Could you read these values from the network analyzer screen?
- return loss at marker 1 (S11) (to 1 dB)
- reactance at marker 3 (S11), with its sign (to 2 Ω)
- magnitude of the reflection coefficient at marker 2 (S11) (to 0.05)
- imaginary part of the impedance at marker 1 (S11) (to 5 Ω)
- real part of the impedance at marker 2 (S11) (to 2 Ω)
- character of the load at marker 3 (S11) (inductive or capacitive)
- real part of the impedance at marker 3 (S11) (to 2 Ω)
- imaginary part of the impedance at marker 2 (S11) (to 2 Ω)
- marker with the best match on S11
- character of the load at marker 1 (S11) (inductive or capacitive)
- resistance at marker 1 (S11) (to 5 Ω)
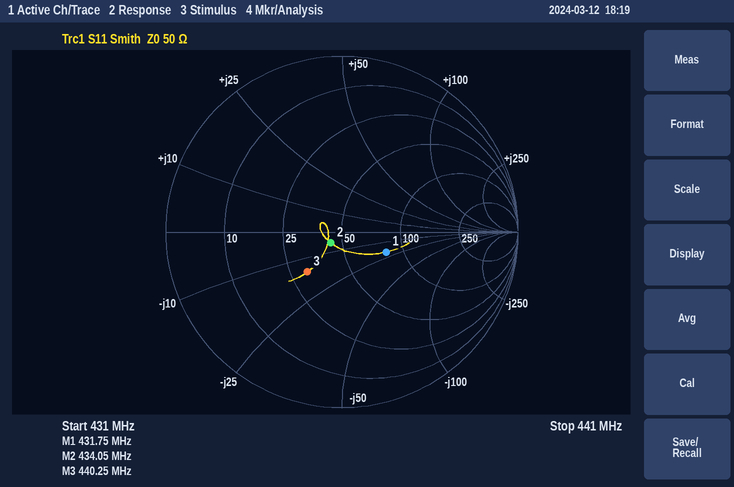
11 dB
-16 Ω
0.10
-20 Ω
44 Ω
capacitive
30 Ω
-6 Ω
marker 2
capacitive
80 Ω
